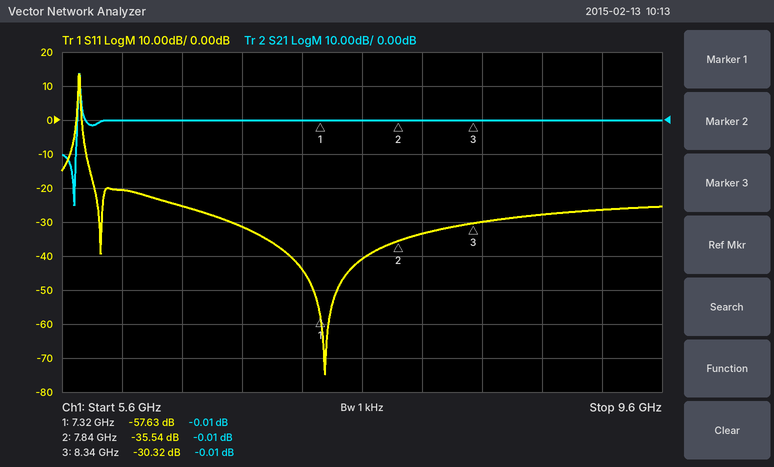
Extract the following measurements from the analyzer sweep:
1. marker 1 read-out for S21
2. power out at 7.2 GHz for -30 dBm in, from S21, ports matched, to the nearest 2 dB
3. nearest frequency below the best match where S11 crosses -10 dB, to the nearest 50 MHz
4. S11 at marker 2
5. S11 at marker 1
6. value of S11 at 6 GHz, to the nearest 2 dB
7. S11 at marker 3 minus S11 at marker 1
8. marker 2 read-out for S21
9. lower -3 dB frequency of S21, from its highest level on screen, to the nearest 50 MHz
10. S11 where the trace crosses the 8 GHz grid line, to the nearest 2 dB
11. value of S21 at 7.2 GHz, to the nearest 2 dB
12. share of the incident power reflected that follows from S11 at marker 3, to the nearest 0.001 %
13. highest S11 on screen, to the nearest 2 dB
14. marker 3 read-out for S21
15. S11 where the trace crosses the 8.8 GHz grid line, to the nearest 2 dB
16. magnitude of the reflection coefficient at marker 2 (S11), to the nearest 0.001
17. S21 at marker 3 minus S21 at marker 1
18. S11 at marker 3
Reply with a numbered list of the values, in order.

1. -0.01 dB
2. -30 dBm
3. 5.75 GHz
4. -35.54 dB
5. -57.63 dB
6. -20 dB
7. 27.31 dB
8. -0.01 dB
9. 5.70 GHz
10. -34 dB
11. 0 dB
12. 0.093 %
13. 14 dB
14. -0.01 dB
15. -28 dB
16. 0.017
17. 0.00 dB
18. -30.32 dB
